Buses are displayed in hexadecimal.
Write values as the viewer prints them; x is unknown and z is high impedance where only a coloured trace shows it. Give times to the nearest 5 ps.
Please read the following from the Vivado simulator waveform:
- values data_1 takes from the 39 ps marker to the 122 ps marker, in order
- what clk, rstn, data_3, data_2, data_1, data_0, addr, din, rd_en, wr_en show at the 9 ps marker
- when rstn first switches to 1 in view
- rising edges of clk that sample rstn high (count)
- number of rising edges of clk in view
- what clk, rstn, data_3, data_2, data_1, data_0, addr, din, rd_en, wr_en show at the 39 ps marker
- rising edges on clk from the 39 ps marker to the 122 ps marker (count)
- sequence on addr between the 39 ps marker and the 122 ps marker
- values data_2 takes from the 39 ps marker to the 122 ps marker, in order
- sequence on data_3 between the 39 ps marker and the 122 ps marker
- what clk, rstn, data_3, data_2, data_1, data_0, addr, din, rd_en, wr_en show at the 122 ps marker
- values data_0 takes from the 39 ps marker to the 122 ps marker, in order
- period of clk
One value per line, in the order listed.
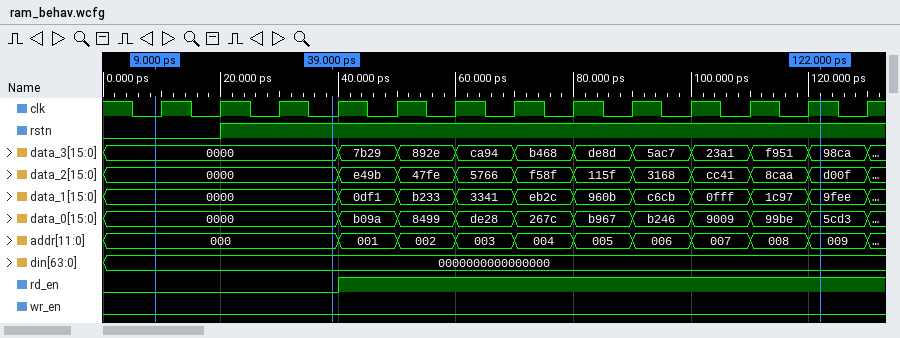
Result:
0000, 0df1, b233, 3341, eb2c, 960b, c6cb, 0fff, 1c97, 9fee
clk=0, rstn=0, data_3=0000, data_2=0000, data_1=0000, data_0=0000, addr=000, din=0000000000000000, rd_en=0, wr_en=0
20 ps
11
13
clk=0, rstn=1, data_3=0000, data_2=0000, data_1=0000, data_0=0000, addr=000, din=0000000000000000, rd_en=0, wr_en=0
9
000, 001, 002, 003, 004, 005, 006, 007, 008, 009
0000, e49b, 47fe, 5766, f58f, 115f, 3168, cc41, 8caa, d00f
0000, 7b29, 892e, ca94, b468, de8d, 5ac7, 23a1, f951, 98ca
clk=1, rstn=1, data_3=98ca, data_2=d00f, data_1=9fee, data_0=5cd3, addr=009, din=0000000000000000, rd_en=1, wr_en=0
0000, b09a, 8499, de28, 267c, b967, b246, 9009, 99be, 5cd3
10 ps
